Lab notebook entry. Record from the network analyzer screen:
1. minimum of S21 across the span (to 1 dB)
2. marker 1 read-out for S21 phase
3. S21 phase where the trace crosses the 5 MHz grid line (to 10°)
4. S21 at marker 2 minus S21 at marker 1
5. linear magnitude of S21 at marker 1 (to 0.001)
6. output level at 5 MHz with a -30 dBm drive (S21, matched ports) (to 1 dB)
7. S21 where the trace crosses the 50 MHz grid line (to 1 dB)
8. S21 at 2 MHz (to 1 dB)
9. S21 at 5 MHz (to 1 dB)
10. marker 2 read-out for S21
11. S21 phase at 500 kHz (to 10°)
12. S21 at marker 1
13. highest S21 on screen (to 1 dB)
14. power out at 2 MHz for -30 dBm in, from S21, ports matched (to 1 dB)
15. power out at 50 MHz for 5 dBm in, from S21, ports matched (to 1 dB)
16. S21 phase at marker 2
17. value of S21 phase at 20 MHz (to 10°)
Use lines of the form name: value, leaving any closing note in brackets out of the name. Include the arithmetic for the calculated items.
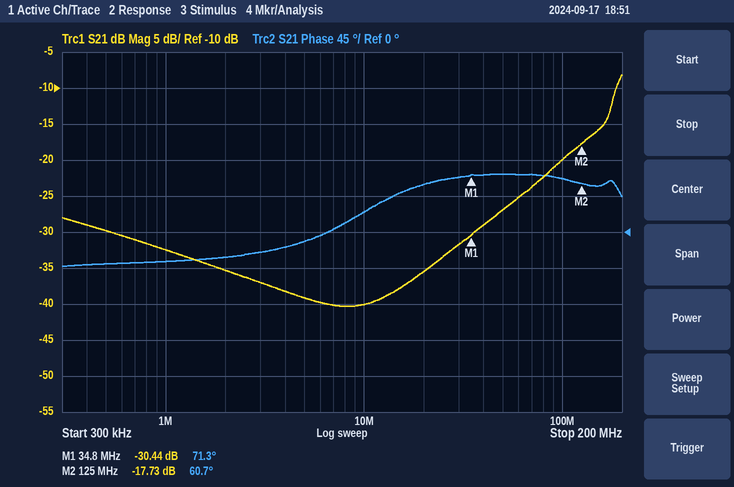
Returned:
minimum of S21 across the span: -40 dB
marker 1 read-out for S21 phase: 71.3°
S21 phase where the trace crosses the 5 MHz grid line: -10°
S21 at marker 2 minus S21 at marker 1: -17.73 − (-30.44) = 12.71 dB
linear magnitude of S21 at marker 1: 10^(-30.44/20) ≈ 0.030
output level at 5 MHz with a -30 dBm drive (S21, matched ports): -30 dBm + (-39 dB) = -69 dBm
S21 where the trace crosses the 50 MHz grid line: -27 dB
S21 at 2 MHz: -35 dB
S21 at 5 MHz: -39 dB
marker 2 read-out for S21: -17.73 dB
S21 phase at 500 kHz: -40°
S21 at marker 1: -30.44 dB
highest S21 on screen: -8 dB
power out at 2 MHz for -30 dBm in, from S21, ports matched: -30 dBm + (-35 dB) = -65 dBm
power out at 50 MHz for 5 dBm in, from S21, ports matched: 5 dBm + (-27 dB) = -22 dBm
S21 phase at marker 2: 60.7°
value of S21 phase at 20 MHz: 60°
